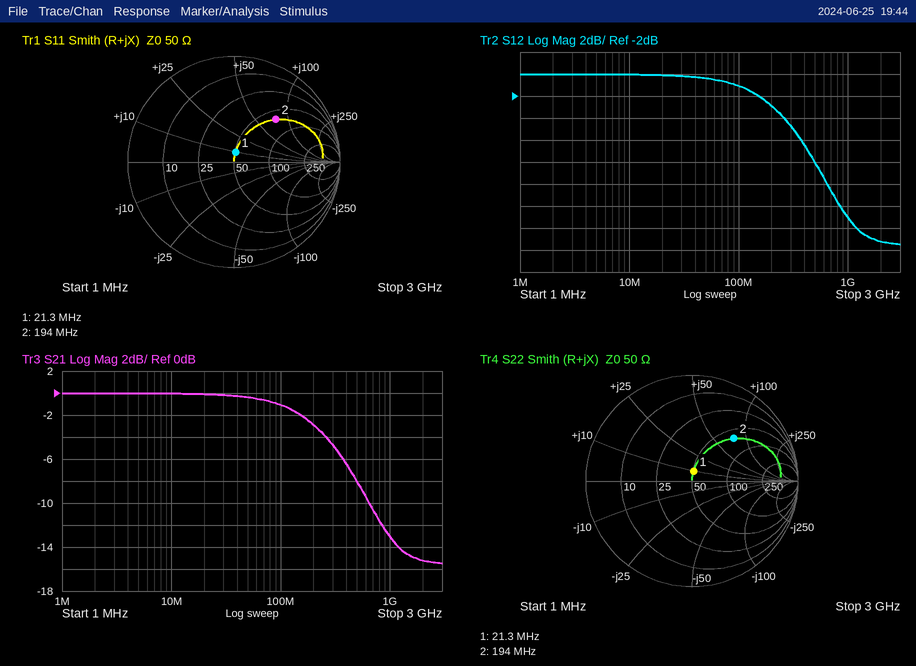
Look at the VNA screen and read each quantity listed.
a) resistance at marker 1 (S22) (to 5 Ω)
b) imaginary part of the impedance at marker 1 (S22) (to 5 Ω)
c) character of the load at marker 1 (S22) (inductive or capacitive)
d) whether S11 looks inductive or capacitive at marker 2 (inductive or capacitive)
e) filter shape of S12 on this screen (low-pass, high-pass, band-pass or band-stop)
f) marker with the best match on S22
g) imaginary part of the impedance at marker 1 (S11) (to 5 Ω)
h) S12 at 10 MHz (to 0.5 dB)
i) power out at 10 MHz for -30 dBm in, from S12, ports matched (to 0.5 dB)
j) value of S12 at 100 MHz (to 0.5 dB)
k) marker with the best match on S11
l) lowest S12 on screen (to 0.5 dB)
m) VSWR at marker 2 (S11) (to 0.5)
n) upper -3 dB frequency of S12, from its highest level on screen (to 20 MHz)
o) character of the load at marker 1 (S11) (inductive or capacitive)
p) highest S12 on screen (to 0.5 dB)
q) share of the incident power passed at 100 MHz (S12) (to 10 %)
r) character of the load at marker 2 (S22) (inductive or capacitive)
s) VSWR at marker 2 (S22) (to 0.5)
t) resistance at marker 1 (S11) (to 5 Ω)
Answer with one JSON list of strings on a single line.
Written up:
["50 Ω", "+10 Ω", "inductive", "inductive", "low-pass", "marker 1", "+10 Ω", "0.0 dB", "-30.0 dBm", "-1.0 dB", "marker 1", "-15.5 dB", "3.5", "200 MHz", "inductive", "0.0 dB", "80 %", "inductive", "3.5", "50 Ω"]
